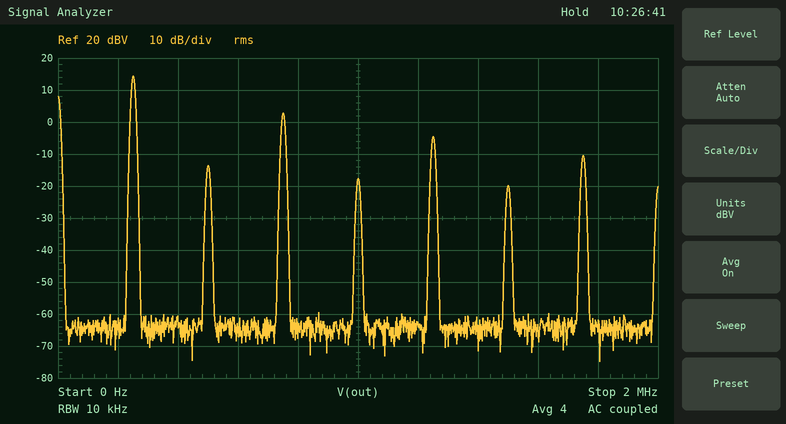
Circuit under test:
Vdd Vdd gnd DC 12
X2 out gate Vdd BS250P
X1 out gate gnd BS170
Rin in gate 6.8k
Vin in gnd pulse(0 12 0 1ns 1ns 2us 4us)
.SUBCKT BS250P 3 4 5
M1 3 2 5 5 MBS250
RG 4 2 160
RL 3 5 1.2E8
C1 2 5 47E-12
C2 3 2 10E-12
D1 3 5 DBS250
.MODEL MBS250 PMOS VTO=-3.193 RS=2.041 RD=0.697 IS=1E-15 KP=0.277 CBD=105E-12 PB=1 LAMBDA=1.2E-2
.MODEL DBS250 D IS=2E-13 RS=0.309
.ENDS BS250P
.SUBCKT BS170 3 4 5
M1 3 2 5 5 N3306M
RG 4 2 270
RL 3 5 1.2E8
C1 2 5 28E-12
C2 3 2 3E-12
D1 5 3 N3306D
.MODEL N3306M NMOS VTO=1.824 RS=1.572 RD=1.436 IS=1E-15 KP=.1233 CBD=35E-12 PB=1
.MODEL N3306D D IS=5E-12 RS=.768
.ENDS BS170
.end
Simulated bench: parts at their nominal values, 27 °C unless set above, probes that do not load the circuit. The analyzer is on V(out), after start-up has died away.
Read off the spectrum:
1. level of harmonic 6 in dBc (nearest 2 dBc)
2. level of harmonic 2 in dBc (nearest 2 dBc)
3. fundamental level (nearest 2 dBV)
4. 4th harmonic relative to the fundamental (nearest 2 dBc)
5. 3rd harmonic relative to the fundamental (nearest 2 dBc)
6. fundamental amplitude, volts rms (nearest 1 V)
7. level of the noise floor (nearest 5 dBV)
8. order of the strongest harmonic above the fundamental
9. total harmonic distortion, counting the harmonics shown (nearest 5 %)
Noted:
-34 dBc
-28 dBc
14 dBV
-32 dBc
-12 dBc
5 V
-65 dBV
3
30 %
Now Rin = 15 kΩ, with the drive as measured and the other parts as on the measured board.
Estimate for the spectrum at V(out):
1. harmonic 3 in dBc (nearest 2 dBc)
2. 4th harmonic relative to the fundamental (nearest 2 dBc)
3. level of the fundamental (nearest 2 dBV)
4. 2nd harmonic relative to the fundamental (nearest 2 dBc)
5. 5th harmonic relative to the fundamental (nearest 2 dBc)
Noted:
-16 dBc
-26 dBc
14 dBV
-24 dBc
-26 dBc
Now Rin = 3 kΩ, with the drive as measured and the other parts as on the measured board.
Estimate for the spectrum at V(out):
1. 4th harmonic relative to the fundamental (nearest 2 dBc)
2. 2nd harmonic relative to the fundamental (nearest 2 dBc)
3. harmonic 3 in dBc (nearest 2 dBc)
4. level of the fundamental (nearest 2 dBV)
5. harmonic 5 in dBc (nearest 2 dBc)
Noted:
-34 dBc
-34 dBc
-10 dBc
14 dBV
-16 dBc
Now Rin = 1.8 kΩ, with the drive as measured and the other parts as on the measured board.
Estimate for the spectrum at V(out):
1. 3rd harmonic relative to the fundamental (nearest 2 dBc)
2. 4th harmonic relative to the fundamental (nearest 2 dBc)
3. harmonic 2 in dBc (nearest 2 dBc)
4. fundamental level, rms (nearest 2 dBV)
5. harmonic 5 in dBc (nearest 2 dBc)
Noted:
-10 dBc
-38 dBc
-38 dBc
14 dBV
-14 dBc
